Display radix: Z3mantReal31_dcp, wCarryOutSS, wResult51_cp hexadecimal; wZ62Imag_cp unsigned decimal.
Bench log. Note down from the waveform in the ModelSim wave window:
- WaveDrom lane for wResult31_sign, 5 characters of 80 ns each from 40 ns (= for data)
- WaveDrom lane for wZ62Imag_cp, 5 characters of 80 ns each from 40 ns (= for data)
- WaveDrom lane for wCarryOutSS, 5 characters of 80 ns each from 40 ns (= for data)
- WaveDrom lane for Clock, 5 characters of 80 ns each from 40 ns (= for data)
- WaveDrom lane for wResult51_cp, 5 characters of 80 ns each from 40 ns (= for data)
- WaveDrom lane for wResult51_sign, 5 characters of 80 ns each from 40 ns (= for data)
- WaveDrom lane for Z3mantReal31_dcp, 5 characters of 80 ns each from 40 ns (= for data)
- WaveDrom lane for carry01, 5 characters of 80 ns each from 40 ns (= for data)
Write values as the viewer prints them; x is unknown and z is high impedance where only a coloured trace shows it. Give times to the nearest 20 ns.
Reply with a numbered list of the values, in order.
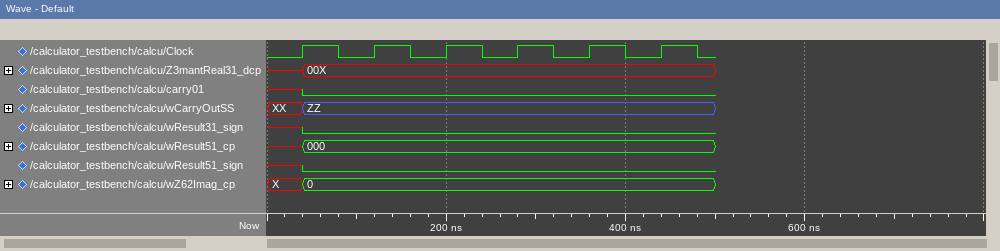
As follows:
1. {name: 'wResult31_sign', wave: '0....'}
2. {name: 'wZ62Imag_cp', wave: '=....', data: '0'}
3. {name: 'wCarryOutSS', wave: '=....', data: 'ZZ'}
4. {name: 'Clock', wave: 'p....'}
5. {name: 'wResult51_cp', wave: '=....', data: '000'}
6. {name: 'wResult51_sign', wave: '0....'}
7. {name: 'Z3mantReal31_dcp', wave: '=....', data: '00X'}
8. {name: 'carry01', wave: '0....'}
